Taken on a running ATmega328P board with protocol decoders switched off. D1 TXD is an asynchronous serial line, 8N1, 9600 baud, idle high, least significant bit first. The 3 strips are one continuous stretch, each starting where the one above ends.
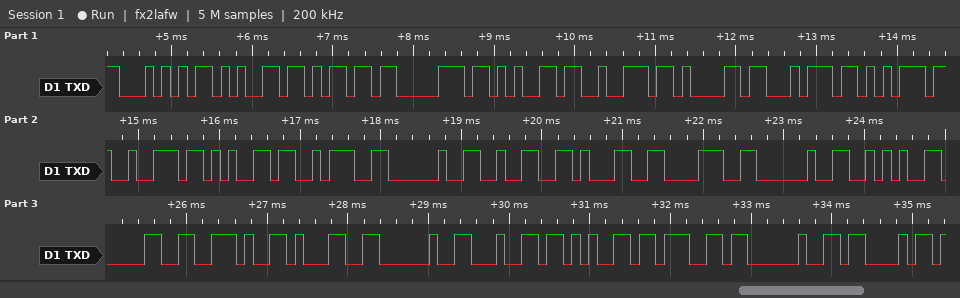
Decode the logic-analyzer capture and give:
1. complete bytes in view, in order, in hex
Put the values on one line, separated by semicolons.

54 65 6D 70 65 72 61 74 75 72 65 3A 20 32 31 38 20 2A 30 2E 31 20 64 65 67 20 43
